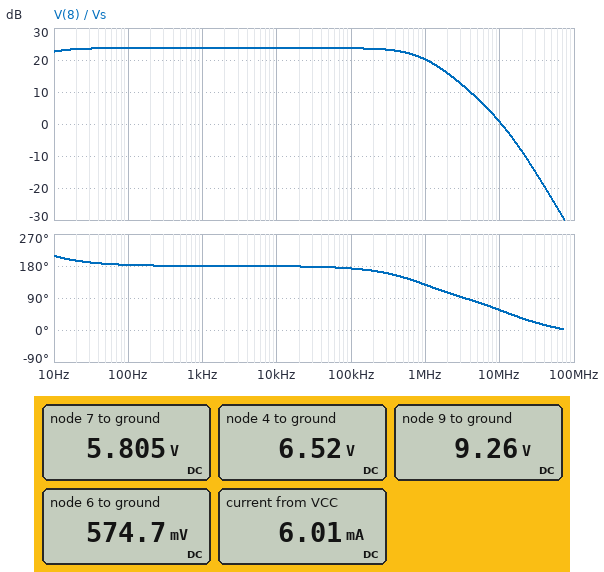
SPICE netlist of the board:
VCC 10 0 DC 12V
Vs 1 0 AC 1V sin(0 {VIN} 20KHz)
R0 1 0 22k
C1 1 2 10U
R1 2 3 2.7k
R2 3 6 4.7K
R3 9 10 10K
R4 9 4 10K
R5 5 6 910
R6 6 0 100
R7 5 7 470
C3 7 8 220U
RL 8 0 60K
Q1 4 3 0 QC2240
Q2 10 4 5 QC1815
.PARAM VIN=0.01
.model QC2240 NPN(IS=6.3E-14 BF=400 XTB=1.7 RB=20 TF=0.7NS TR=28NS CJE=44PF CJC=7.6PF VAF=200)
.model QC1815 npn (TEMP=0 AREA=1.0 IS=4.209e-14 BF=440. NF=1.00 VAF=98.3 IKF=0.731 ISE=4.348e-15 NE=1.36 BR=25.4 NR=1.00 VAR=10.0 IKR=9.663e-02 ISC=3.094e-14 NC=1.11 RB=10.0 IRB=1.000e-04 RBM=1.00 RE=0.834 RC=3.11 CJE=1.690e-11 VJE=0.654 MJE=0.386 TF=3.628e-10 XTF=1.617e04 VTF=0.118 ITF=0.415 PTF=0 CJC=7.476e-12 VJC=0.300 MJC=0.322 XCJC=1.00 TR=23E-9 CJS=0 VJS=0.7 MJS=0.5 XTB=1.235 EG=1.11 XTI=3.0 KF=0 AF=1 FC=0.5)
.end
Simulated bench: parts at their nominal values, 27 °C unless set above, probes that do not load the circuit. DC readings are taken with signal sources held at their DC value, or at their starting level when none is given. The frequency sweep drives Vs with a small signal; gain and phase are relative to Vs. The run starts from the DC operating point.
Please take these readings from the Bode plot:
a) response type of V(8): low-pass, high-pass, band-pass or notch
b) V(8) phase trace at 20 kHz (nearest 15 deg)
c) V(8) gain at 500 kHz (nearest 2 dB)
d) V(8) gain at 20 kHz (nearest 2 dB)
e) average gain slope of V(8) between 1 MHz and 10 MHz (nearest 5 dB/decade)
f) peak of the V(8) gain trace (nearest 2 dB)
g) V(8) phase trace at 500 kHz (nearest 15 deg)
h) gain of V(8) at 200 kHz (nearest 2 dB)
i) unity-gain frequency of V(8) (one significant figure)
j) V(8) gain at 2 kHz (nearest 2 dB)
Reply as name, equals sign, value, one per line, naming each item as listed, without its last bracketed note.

response type of V(8): low-pass, high-pass, band-pass or notch = low-pass
V(8) phase trace at 20 kHz = 180 deg
V(8) gain at 500 kHz = 22 dB
V(8) gain at 20 kHz = 24 dB
average gain slope of V(8) between 1 MHz and 10 MHz = -20 dB/decade
peak of the V(8) gain trace = 24 dB
V(8) phase trace at 500 kHz = 150 deg
gain of V(8) at 200 kHz = 24 dB
unity-gain frequency of V(8) = 10 MHz
V(8) gain at 2 kHz = 24 dB
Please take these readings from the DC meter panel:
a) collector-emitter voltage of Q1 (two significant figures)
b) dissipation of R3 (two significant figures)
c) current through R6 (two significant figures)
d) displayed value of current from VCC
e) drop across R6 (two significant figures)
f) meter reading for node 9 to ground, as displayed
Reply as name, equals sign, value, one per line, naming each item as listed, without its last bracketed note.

collector-emitter voltage of Q1 = 6.5 V
dissipation of R3 = 750 µW
current through R6 = 5.7 mA
displayed value of current from VCC = 6.01 mA
drop across R6 = 570 mV
meter reading for node 9 to ground, as displayed = 9.26 V
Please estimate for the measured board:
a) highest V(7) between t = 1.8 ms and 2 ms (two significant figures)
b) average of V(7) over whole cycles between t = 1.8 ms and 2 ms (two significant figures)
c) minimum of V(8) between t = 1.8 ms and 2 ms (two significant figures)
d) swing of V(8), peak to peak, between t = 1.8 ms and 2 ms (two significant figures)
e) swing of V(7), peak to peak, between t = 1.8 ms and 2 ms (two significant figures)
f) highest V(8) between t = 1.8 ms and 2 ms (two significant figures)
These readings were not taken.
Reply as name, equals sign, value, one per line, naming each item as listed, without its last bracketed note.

highest V(7) between t = 1.8 ms and 2 ms = 6.0 V
average of V(7) over whole cycles between t = 1.8 ms and 2 ms = 5.8 V
minimum of V(8) between t = 1.8 ms and 2 ms = -150 mV
swing of V(8), peak to peak, between t = 1.8 ms and 2 ms = 310 mV
swing of V(7), peak to peak, between t = 1.8 ms and 2 ms = 310 mV
highest V(8) between t = 1.8 ms and 2 ms = 150 mV
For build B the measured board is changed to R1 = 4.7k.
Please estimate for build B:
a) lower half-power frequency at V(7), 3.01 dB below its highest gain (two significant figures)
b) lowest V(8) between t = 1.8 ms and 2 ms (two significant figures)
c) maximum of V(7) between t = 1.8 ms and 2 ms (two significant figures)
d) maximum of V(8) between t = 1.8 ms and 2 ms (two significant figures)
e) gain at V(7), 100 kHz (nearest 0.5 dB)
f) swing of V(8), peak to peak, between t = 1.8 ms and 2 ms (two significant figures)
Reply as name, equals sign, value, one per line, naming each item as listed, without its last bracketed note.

lower half-power frequency at V(7), 3.01 dB below its highest gain = 3.2 Hz
lowest V(8) between t = 1.8 ms and 2 ms = -91 mV
maximum of V(7) between t = 1.8 ms and 2 ms = 5.9 V
maximum of V(8) between t = 1.8 ms and 2 ms = 91 mV
gain at V(7), 100 kHz = 19.0 dB
swing of V(8), peak to peak, between t = 1.8 ms and 2 ms = 180 mV
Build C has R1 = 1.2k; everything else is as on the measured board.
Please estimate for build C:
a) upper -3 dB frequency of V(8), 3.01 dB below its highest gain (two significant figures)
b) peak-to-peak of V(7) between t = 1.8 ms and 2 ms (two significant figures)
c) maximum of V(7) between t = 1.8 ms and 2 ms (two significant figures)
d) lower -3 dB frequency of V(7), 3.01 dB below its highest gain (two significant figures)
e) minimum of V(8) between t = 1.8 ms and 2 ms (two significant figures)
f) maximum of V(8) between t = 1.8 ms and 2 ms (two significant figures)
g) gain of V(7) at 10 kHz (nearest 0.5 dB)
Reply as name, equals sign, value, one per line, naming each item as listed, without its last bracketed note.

upper -3 dB frequency of V(8), 3.01 dB below its highest gain = 900 kHz
peak-to-peak of V(7) between t = 1.8 ms and 2 ms = 620 mV
maximum of V(7) between t = 1.8 ms and 2 ms = 6.1 V
lower -3 dB frequency of V(7), 3.01 dB below its highest gain = 11 Hz
minimum of V(8) between t = 1.8 ms and 2 ms = -310 mV
maximum of V(8) between t = 1.8 ms and 2 ms = 310 mV
gain of V(7) at 10 kHz = 30.0 dB
